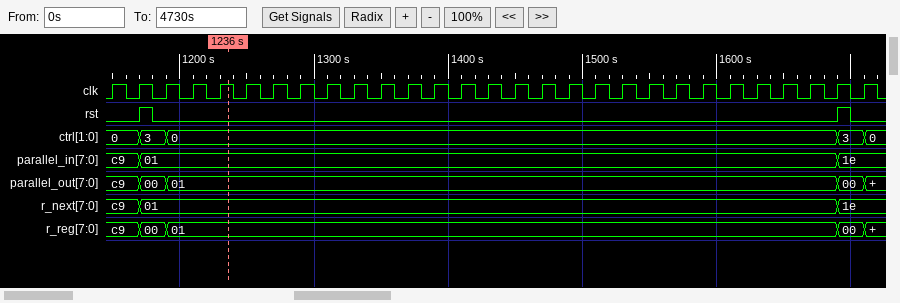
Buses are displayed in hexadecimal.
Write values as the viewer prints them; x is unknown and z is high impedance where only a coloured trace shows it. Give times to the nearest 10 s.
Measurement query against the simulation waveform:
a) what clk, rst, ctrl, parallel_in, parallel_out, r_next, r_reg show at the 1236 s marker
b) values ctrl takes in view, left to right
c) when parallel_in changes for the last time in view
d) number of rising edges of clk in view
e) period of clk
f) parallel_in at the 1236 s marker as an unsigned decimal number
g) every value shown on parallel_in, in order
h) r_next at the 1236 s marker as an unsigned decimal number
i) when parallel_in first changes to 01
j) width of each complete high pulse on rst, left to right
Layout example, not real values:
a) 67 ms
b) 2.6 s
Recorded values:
a) clk=1, rst=0, ctrl=0, parallel_in=01, parallel_out=01, r_next=01, r_reg=01
b) 0, 3, 0, 3, 0
c) 1690 s
d) 29
e) 20 s
f) 1
g) c9, 01, 1e
h) 1
i) 1170 s
j) 10 s, 10 s
